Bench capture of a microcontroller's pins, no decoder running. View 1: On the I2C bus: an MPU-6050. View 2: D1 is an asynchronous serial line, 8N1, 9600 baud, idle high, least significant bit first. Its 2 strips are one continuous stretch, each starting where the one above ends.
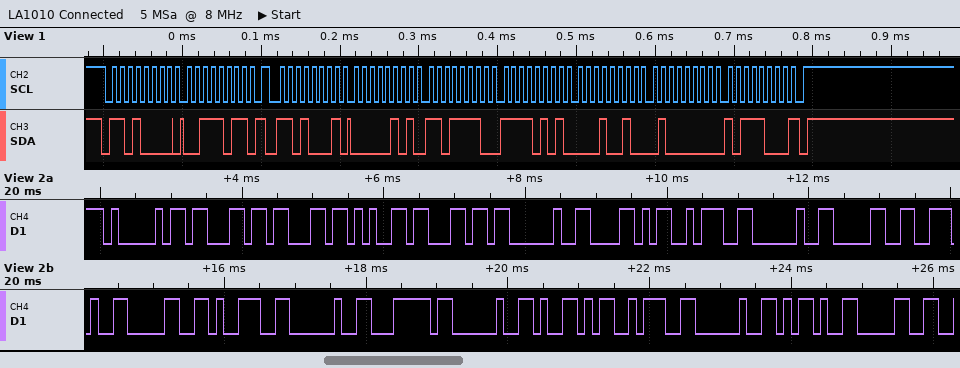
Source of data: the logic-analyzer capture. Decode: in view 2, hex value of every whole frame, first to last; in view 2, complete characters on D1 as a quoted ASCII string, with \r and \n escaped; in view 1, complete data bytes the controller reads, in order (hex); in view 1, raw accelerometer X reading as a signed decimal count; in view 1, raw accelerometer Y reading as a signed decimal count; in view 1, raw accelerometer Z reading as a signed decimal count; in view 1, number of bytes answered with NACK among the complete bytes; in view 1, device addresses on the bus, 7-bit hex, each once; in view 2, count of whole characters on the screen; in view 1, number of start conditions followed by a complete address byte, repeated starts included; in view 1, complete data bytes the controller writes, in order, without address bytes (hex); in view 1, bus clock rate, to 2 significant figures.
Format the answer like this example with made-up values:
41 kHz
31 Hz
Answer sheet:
41 63 63 65 6C 20 58 3A 20 30 2E 30 39 20 7C 20 59 3A 20 2D 30
"Accel X: 0.09 | Y: -0"
05 DE F5 12 40 B8
1502
-2798
16568
1
0x68
21
2
3B
100 kHz
